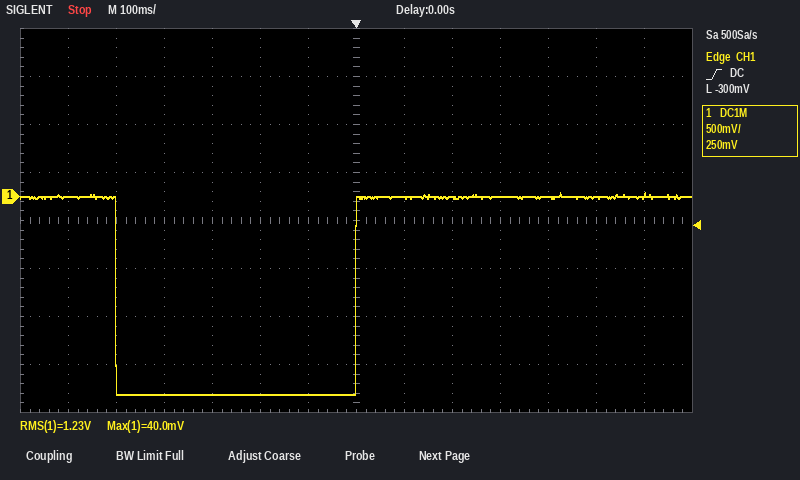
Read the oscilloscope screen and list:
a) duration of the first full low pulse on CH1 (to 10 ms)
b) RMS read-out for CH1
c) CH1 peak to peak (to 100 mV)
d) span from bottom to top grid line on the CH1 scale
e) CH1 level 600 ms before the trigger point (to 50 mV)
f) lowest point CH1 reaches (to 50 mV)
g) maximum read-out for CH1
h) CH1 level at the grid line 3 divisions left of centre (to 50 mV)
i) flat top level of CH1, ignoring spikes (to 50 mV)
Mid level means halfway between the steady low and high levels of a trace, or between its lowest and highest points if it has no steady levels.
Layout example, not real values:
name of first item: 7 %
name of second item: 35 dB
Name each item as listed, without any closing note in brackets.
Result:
duration of the first full low pulse on CH1: 500 ms
RMS read-out for CH1: 1.23 V
CH1 peak to peak: 2.10 V
span from bottom to top grid line on the CH1 scale: 4 V
CH1 level 600 ms before the trigger point: 0 mV
lowest point CH1 reaches: -2.05 V
maximum read-out for CH1: 40.0 mV
CH1 level at the grid line 3 divisions left of centre: -2.05 V
flat top level of CH1, ignoring spikes: 0 mV
